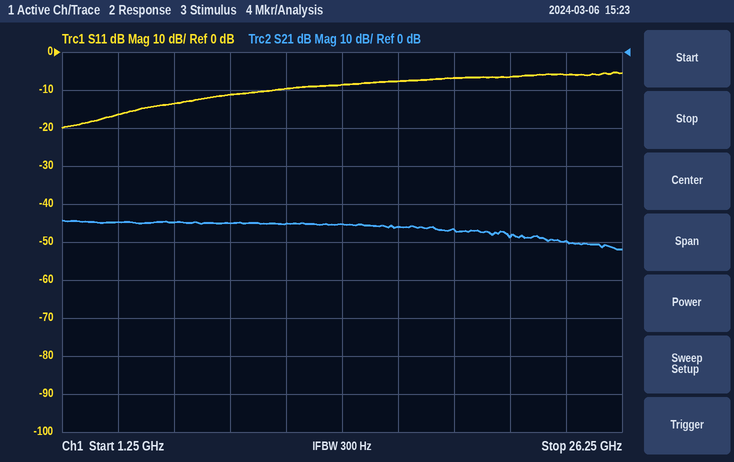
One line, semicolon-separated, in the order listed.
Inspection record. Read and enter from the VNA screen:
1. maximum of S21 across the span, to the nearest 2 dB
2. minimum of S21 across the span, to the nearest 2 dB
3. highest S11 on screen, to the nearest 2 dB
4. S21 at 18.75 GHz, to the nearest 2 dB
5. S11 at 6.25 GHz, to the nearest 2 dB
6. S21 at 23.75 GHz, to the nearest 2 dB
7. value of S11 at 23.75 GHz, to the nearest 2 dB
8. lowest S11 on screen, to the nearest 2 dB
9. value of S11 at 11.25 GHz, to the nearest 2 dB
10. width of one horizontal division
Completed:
-44 dB; -52 dB; -6 dB; -46 dB; -14 dB; -50 dB; -6 dB; -20 dB; -10 dB; 2.5 GHz
